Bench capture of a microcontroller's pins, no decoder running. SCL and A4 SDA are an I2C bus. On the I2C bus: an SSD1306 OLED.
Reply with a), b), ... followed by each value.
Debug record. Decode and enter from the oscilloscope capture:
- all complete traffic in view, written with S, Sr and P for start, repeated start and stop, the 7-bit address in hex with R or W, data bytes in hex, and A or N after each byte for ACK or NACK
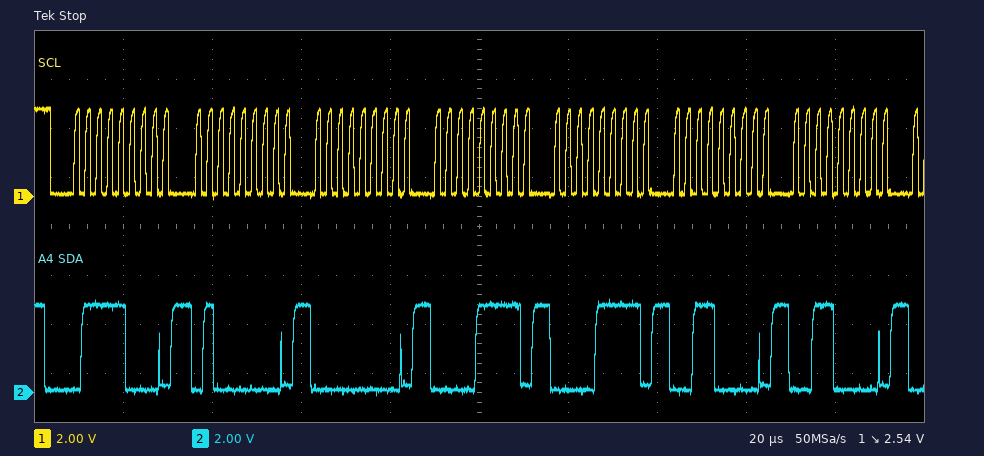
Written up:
a) S 3CW A 40 A 00 A 0F A 0F A 30 A 30 A
